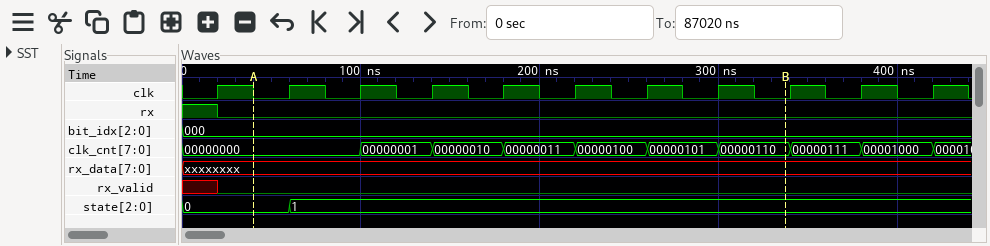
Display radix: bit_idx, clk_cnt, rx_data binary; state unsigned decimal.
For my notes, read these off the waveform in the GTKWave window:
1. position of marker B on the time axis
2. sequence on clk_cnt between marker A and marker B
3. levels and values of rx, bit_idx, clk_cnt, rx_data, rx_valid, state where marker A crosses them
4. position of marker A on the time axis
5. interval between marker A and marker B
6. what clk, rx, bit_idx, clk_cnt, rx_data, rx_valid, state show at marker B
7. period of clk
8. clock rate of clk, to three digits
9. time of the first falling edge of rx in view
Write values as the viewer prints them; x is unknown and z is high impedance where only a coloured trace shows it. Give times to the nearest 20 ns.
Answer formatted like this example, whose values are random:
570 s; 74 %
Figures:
340 ns; 00000000, 00000001, 00000010, 00000011, 00000100, 00000101, 00000110; rx=0, bit_idx=000, clk_cnt=00000000, rx_data=xxxxxxxx, rx_valid=0, state=0; 40 ns; 300 ns; clk=0, rx=0, bit_idx=000, clk_cnt=00000110, rx_data=xxxxxxxx, rx_valid=0, state=1; 40 ns; 25.0 MHz; 20 ns
